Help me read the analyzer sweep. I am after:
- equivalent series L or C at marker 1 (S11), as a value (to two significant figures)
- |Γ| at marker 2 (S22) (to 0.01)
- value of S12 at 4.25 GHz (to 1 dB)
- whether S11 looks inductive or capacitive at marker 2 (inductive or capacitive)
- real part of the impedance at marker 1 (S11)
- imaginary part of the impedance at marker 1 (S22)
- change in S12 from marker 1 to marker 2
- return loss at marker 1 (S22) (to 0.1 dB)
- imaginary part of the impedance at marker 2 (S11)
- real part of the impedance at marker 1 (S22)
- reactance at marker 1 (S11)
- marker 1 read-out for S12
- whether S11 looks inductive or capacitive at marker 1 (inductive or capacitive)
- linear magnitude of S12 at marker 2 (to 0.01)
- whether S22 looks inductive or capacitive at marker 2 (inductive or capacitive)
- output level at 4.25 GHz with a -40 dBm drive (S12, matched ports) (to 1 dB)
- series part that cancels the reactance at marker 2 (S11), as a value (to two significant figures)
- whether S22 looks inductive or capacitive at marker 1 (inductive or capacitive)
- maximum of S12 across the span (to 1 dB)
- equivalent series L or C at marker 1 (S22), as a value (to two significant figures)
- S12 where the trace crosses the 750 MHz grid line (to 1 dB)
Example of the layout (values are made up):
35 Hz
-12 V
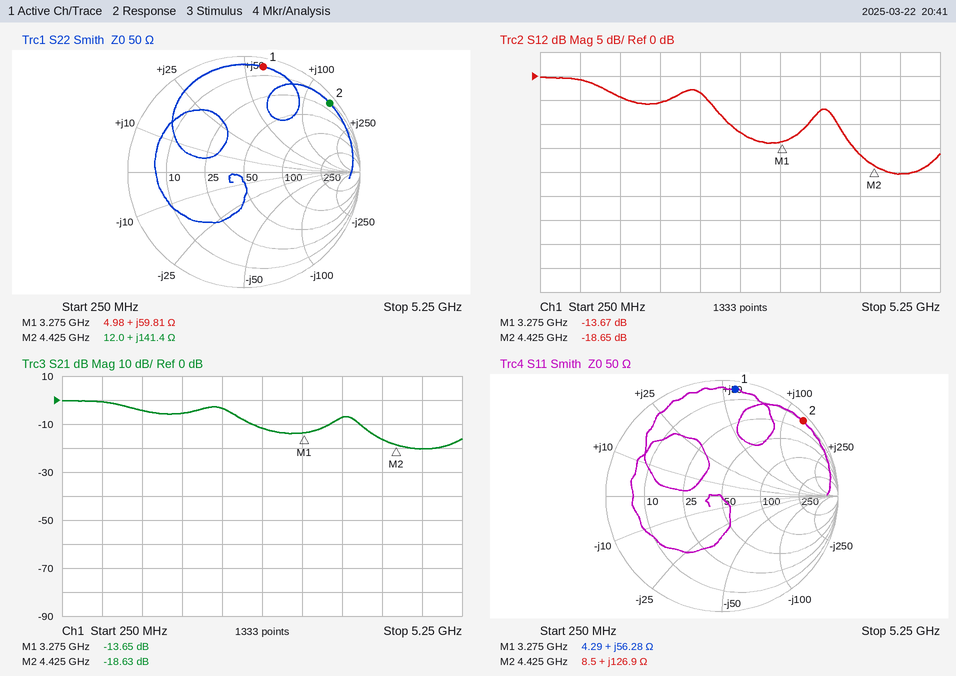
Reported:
2.7 nH
0.95
-16 dB
inductive
4.29 Ω
+59.81 Ω
-4.98 dB
0.7 dB
+126.9 Ω
4.98 Ω
+56.28 Ω
-13.67 dB
inductive
0.12
inductive
-56 dBm
280 fF
inductive
0 dB
2.9 nH
-1 dB
